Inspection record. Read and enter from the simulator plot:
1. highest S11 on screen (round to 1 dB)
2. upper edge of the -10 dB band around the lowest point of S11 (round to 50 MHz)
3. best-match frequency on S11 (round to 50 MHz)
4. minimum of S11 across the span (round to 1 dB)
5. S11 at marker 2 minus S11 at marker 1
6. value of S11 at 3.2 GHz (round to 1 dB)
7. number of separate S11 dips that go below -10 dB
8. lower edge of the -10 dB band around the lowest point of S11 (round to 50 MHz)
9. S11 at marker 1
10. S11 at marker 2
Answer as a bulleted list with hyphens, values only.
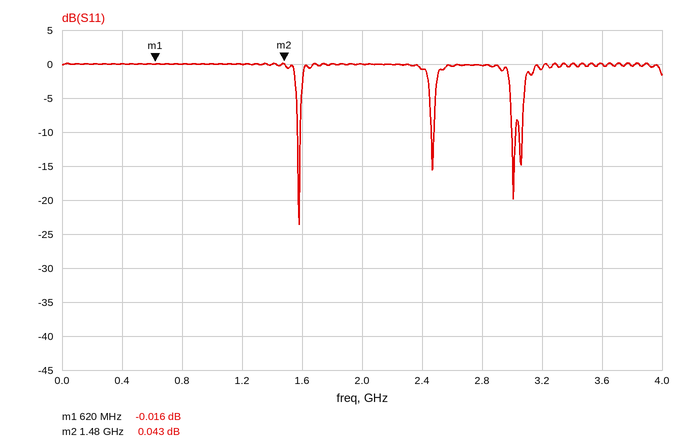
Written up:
- 0 dB
- 1.60 GHz
- 1.60 GHz
- -24 dB
- 0.059 dB
- -1 dB
- 4
- 1.55 GHz
- -0.016 dB
- 0.043 dB
